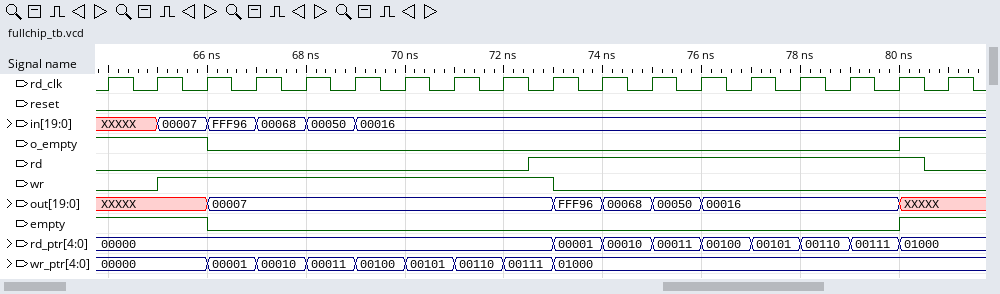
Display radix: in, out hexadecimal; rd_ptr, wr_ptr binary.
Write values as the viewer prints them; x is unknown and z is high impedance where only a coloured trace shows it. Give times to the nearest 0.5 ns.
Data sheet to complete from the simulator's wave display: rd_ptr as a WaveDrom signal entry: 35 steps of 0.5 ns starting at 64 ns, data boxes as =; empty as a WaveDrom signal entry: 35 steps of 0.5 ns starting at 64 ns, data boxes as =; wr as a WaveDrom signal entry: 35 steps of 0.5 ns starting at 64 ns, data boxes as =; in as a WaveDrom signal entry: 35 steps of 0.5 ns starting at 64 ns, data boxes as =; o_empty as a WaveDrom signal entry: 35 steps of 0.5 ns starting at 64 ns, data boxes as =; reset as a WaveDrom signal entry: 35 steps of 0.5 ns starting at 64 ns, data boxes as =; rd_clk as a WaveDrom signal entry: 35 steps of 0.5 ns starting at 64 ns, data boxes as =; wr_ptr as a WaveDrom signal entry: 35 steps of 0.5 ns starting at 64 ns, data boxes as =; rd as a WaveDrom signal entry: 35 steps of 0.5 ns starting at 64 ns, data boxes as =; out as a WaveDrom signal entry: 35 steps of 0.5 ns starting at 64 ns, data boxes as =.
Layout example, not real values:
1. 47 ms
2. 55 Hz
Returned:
1. {name: 'rd_ptr', wave: '=.................=.=.=.=.=.=.=.=..', data: '00000 00001 00010 00011 00100 00101 00110 00111 01000'}
2. {name: 'empty', wave: '1...0...........................1..'}
3. {name: 'wr', wave: '0.1...............0................'}
4. {name: 'in', wave: 'x.=.=.=.=.=........................', data: '00007 FFF96 00068 00050 00016'}
5. {name: 'o_empty', wave: '1...0...........................1..'}
6. {name: 'reset', wave: '0..................................'}
7. {name: 'rd_clk', wave: '10101010101010101010101010101010101'}
8. {name: 'wr_ptr', wave: '=...=.=.=.=.=.=.=.=................', data: '00000 00001 00010 00011 00100 00101 00110 00111 01000'}
9. {name: 'rd', wave: '0................1...............0.'}
10. {name: 'out', wave: 'x...=.............=.=.=.=.......x..', data: '00007 FFF96 00068 00050 00016'}
